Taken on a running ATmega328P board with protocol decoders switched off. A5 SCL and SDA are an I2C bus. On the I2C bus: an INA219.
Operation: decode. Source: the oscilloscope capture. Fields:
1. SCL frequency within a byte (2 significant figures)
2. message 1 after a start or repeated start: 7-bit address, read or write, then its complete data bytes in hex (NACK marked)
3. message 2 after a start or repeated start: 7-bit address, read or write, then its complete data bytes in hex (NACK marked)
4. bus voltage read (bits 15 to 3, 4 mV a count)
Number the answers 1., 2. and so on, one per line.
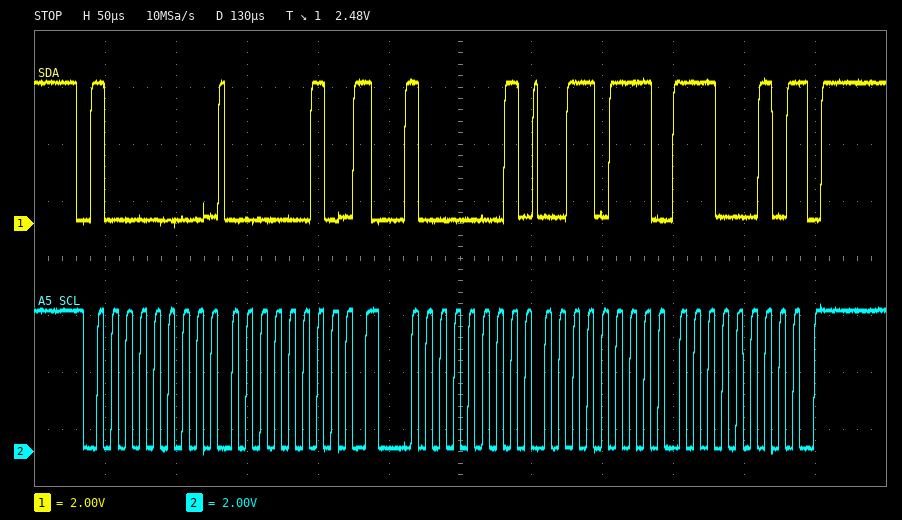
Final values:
1. 100 kHz
2. 0x40 write: 02
3. 0x40 read: 37 E2 NACK
4. 7.152 V
